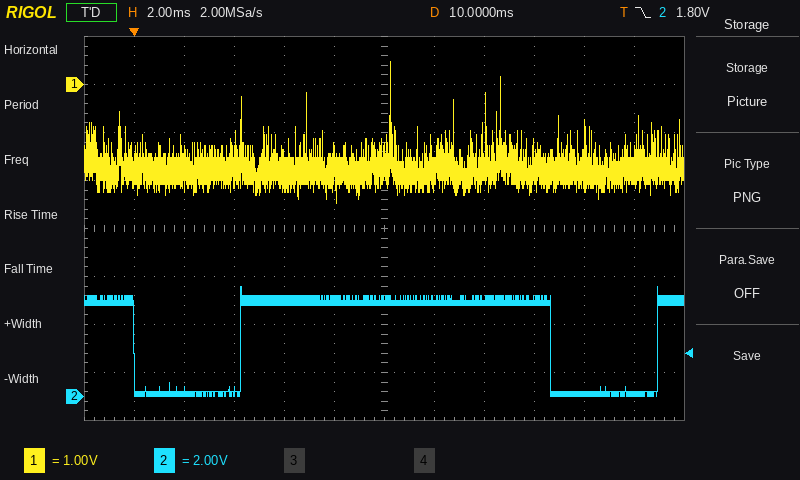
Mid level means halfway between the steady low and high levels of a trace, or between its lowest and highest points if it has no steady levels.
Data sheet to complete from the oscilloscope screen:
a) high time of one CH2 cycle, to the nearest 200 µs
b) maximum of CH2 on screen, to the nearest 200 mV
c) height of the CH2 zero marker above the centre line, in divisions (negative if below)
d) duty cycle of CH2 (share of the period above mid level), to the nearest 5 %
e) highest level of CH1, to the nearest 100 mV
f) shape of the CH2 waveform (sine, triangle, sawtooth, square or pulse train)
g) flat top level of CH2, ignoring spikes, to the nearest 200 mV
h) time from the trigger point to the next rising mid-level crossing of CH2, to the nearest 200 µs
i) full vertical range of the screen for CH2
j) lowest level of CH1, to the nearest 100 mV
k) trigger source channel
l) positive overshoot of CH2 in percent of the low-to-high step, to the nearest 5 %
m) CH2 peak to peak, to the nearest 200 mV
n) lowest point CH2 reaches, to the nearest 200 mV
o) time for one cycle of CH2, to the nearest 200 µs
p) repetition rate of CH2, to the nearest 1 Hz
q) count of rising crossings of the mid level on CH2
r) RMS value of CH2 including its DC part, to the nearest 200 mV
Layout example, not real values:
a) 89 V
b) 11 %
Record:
a) 12.4 ms
b) 4.6 V
c) -3.5 div
d) 75 %
e) 500 mV
f) pulse train
g) 4.0 V
h) 4.2 ms
i) 16 V
j) -2.5 V
k) CH2
l) 15 %
m) 4.6 V
n) 0.0 V
o) 16.6 ms
p) 60 Hz
q) 2
r) 3.4 V
